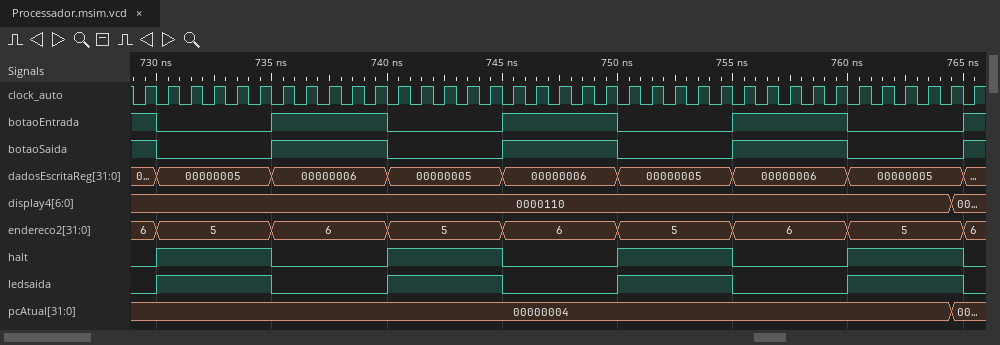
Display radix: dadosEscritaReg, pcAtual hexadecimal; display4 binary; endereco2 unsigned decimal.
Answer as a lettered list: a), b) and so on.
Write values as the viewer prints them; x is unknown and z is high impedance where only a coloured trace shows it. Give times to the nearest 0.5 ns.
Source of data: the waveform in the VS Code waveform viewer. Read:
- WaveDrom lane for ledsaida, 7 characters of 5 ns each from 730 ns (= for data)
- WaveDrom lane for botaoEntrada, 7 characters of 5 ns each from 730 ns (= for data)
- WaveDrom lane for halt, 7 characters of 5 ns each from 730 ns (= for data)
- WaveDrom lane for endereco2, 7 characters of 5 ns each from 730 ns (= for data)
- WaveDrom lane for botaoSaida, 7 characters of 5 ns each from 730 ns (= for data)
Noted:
a) {name: 'ledsaida', wave: '1010101'}
b) {name: 'botaoEntrada', wave: '0101010'}
c) {name: 'halt', wave: '1010101'}
d) {name: 'endereco2', wave: '=======', data: '5 6 5 6 5 6 5'}
e) {name: 'botaoSaida', wave: '0101010'}
